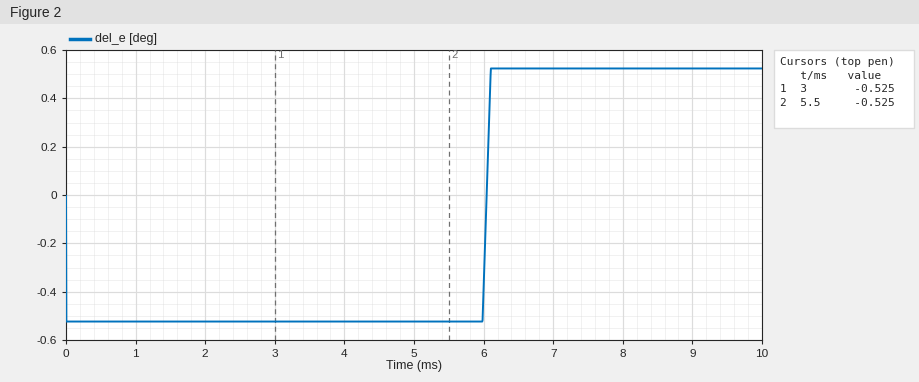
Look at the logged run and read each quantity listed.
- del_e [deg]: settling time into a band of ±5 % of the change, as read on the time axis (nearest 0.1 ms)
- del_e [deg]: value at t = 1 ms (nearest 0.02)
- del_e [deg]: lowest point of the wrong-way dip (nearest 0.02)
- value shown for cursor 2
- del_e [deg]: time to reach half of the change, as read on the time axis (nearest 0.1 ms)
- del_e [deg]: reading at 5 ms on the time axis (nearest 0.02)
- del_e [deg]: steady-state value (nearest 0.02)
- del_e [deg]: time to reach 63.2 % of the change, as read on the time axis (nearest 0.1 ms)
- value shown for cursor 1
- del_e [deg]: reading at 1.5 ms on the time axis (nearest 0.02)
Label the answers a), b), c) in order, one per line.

a) 6.1 ms
b) -0.52
c) -0.52
d) -0.525
e) 6.1 ms
f) -0.52
g) 0.52
h) 6.1 ms
i) -0.525
j) -0.52
